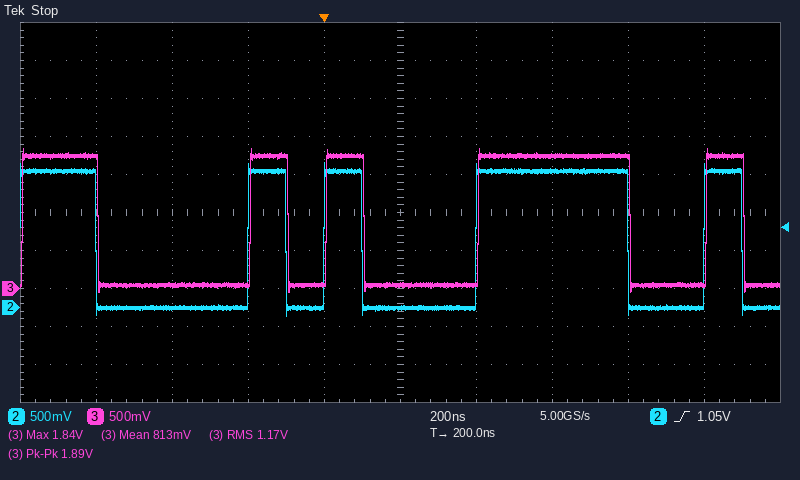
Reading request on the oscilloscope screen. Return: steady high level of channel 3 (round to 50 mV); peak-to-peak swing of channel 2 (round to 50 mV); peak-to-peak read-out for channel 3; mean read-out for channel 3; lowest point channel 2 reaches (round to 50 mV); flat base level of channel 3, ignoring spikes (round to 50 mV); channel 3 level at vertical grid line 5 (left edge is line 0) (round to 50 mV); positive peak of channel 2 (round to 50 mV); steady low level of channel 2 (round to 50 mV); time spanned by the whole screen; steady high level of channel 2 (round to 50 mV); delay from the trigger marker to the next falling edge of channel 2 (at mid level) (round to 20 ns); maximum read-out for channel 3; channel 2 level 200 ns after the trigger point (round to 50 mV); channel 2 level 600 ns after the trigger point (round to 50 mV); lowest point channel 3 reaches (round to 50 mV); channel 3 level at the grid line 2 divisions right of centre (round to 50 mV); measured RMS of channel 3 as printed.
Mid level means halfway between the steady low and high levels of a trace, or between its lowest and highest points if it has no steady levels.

1.75 V
2.00 V
1.89 V
813 mV
-100 mV
50 mV
50 mV
1.90 V
0 mV
2 µs
1.80 V
100 ns
1.84 V
0 mV
1.80 V
-50 mV
1.75 V
1.17 V
